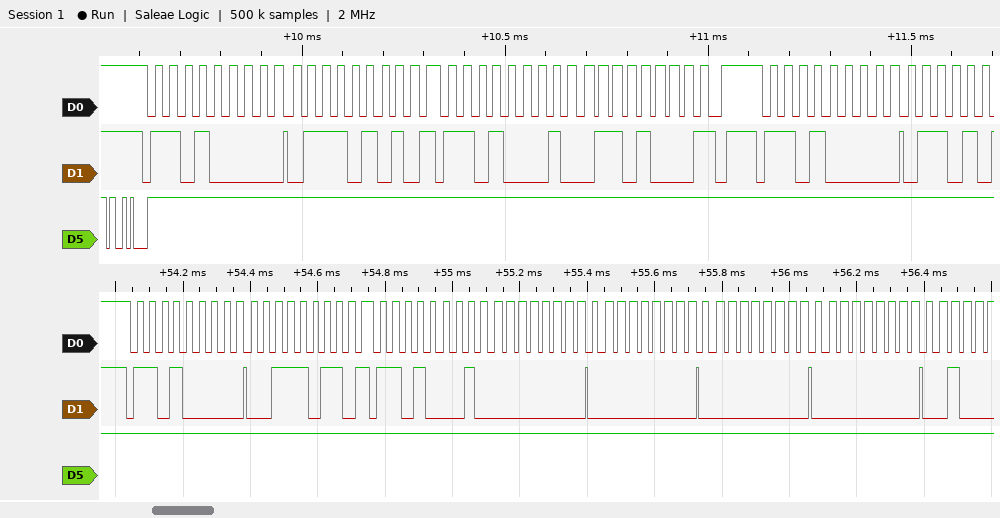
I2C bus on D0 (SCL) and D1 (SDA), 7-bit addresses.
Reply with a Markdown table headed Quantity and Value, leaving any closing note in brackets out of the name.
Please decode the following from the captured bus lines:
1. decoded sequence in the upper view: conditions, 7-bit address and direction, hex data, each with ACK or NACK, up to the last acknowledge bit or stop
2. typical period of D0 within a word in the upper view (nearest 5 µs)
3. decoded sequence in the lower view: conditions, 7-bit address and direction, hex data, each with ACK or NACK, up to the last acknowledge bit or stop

| Quantity | Value |
|---|---|
| decoded sequence in the upper view: conditions, 7-bit address and direction, hex data, each with ACK or NACK, up to the last acknowledge bit or stop | start, address 68 write ACK, 75 ACK, repeated start, address 68 read ACK, 68 NACK, stop, start, address 68 write ACK |
| typical period of D0 within a word in the upper view | 35 µs |
| decoded sequence in the lower view: conditions, 7-bit address and direction, hex data, each with ACK or NACK, up to the last acknowledge bit or stop | start, address 68 write ACK, 3B ACK, repeated start, address 68 read ACK, 00 ACK, 00 ACK, 00 ACK, 00 ACK |
